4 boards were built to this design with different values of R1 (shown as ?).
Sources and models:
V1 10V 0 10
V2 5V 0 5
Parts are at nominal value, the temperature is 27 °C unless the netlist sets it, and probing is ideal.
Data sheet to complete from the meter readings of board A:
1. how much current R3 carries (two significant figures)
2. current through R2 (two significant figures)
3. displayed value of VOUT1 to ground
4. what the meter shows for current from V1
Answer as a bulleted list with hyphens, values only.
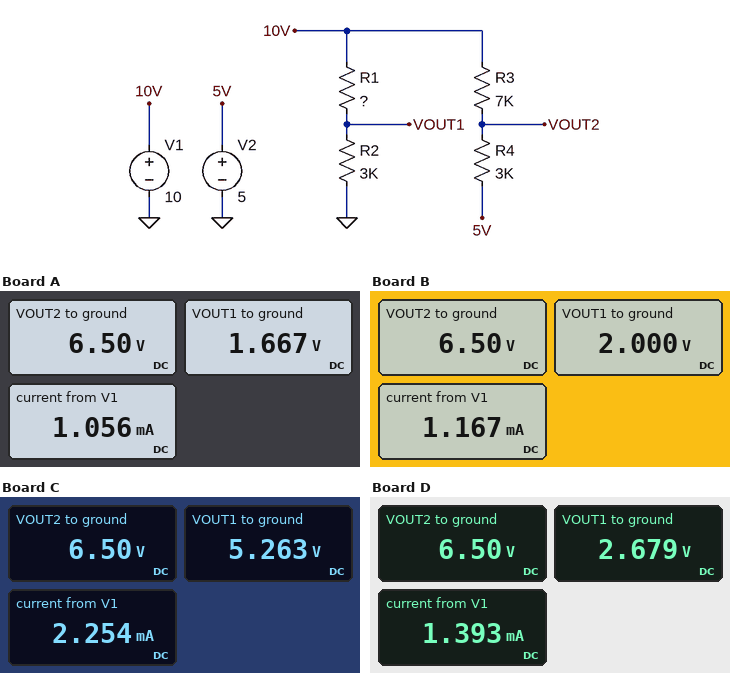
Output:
- 500 µA
- 560 µA
- 1.667 V
- 1.056 mA
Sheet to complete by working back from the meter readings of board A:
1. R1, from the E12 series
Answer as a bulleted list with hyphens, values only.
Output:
- 15 kΩ
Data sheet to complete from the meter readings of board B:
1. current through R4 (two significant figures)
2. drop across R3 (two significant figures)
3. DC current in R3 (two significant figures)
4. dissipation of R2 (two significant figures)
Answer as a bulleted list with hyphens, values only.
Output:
- 500 µA
- 3.5 V
- 500 µA
- 1.3 mW
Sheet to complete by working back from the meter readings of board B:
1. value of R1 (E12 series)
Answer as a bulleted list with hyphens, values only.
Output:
- 12 kΩ
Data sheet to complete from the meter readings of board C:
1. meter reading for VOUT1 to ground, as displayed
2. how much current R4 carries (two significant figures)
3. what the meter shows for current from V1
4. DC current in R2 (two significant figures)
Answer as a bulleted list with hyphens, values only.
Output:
- 5.263 V
- 500 µA
- 2.254 mA
- 1.8 mA
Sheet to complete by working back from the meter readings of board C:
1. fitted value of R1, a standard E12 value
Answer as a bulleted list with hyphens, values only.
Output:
- 2.7 kΩ
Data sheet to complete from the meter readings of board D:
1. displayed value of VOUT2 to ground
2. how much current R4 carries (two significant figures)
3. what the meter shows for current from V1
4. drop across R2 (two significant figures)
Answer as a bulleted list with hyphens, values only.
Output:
- 6.50 V
- 500 µA
- 1.393 mA
- 2.7 V
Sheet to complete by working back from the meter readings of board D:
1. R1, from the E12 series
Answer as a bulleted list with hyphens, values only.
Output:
- 8.2 kΩ
